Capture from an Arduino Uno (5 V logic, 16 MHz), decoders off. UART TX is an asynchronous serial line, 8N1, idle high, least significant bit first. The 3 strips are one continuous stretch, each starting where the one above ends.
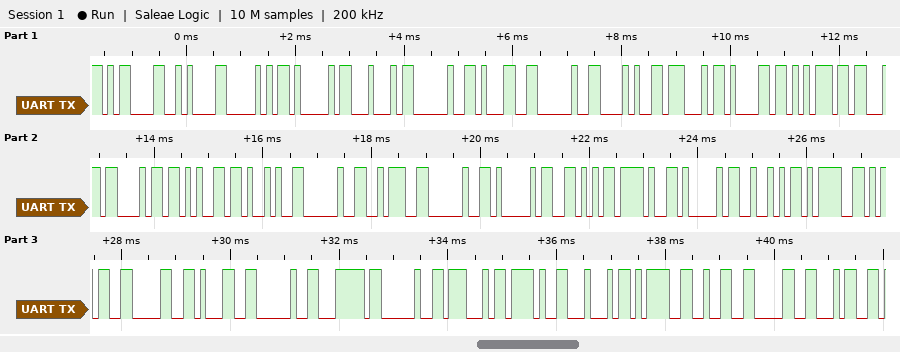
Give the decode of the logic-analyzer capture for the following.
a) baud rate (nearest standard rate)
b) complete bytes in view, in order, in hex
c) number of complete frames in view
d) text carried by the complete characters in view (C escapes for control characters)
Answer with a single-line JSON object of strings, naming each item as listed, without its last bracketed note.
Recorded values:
{"baud rate": "9600 baud", "complete bytes in view, in order, in hex": "0D 0A 50 41 44 20 31 20 28 47 61 75 63 68 65 29 20 3A 20 41 56 2F 41 52 3D 35 30 31 20 7C 20 47 2F 44 3D 32 30 34", "number of complete frames in view": "38", "text carried by the complete characters in view": "\"\\r\\nPAD 1 (Gauche) : AV/AR=501 | G/D=204\""}
